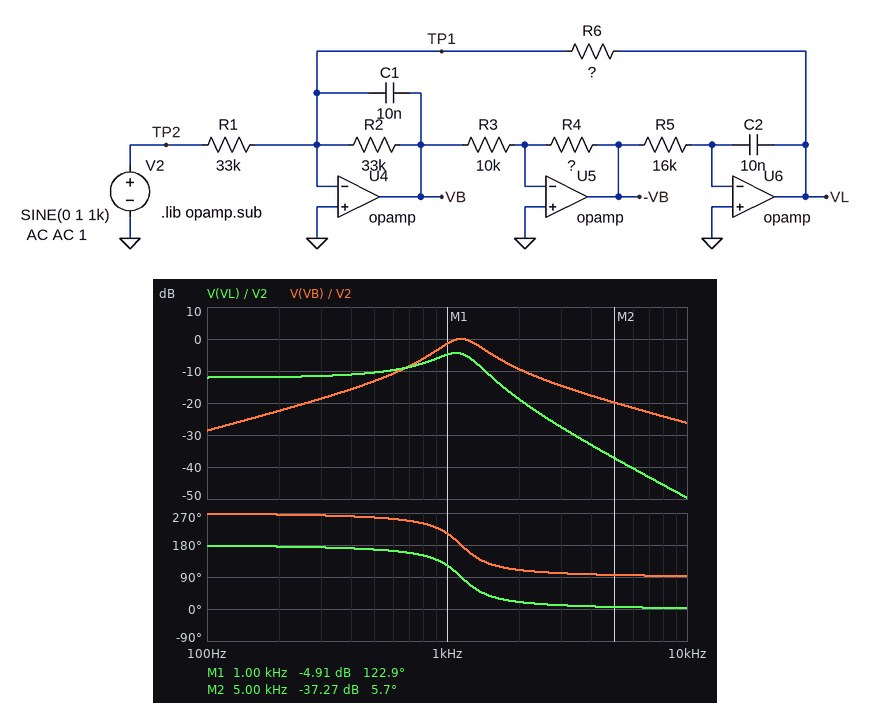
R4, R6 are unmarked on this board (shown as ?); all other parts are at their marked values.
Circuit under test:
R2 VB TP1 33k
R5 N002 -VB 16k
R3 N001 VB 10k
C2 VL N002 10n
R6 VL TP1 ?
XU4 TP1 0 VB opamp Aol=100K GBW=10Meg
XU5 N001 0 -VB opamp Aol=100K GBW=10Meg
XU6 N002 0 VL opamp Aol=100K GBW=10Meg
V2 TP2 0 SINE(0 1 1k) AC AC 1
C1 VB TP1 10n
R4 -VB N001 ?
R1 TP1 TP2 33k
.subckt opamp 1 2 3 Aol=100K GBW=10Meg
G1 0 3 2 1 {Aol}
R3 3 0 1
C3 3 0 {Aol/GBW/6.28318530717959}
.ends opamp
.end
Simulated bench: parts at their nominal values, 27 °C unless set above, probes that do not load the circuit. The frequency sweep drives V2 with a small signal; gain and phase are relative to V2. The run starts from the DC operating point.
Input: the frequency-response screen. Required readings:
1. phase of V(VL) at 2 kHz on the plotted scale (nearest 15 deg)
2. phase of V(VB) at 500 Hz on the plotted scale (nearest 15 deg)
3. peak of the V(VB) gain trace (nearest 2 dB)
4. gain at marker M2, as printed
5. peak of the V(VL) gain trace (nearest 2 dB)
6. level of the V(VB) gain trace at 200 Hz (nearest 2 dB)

15 deg
255 deg
0 dB
-37.27 dB
-4 dB
-22 dB
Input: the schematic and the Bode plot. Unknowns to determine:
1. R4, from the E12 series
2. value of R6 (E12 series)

6.8 kΩ
8.2 kΩ
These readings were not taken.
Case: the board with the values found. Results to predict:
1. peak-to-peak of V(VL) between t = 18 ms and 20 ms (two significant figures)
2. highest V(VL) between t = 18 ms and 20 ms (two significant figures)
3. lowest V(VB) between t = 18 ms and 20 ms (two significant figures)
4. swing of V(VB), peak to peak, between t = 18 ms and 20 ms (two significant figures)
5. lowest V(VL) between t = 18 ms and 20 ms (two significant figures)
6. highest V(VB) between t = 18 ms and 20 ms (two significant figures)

1.1 V
570 mV
-840 mV
1.7 V
-570 mV
840 mV
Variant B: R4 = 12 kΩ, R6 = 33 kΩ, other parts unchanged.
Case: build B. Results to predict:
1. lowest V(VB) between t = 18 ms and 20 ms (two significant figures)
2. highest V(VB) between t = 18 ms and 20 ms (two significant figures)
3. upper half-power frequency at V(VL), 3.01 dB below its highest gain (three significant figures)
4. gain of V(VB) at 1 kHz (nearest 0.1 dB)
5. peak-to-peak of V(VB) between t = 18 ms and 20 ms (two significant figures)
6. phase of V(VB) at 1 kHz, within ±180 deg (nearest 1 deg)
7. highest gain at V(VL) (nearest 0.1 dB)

-750 mV
750 mV
898 Hz
-2.5 dB
1.5 V
139 deg
4.4 dB
